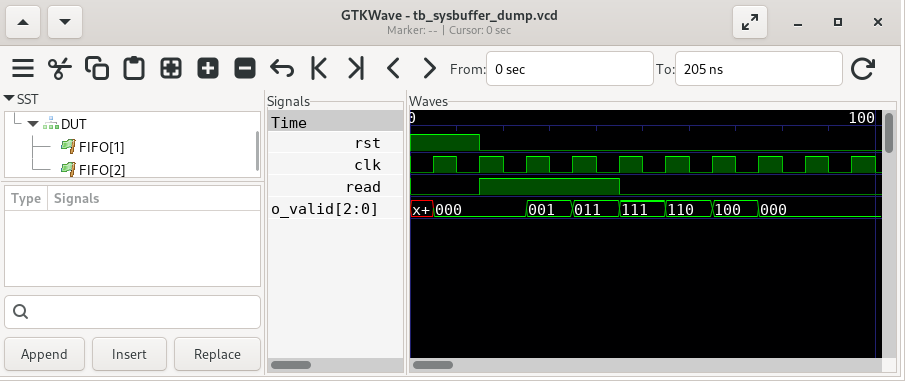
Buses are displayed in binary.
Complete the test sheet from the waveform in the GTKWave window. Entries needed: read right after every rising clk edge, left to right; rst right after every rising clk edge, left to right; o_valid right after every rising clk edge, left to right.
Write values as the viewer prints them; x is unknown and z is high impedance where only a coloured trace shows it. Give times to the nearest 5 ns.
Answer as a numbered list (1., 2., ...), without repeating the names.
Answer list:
1. 0 1 1 1 0 0 0 0 0 0
2. 1 0 0 0 0 0 0 0 0 0
3. 000, 000, 001, 011, 111, 110, 100, 000, 000, 000
